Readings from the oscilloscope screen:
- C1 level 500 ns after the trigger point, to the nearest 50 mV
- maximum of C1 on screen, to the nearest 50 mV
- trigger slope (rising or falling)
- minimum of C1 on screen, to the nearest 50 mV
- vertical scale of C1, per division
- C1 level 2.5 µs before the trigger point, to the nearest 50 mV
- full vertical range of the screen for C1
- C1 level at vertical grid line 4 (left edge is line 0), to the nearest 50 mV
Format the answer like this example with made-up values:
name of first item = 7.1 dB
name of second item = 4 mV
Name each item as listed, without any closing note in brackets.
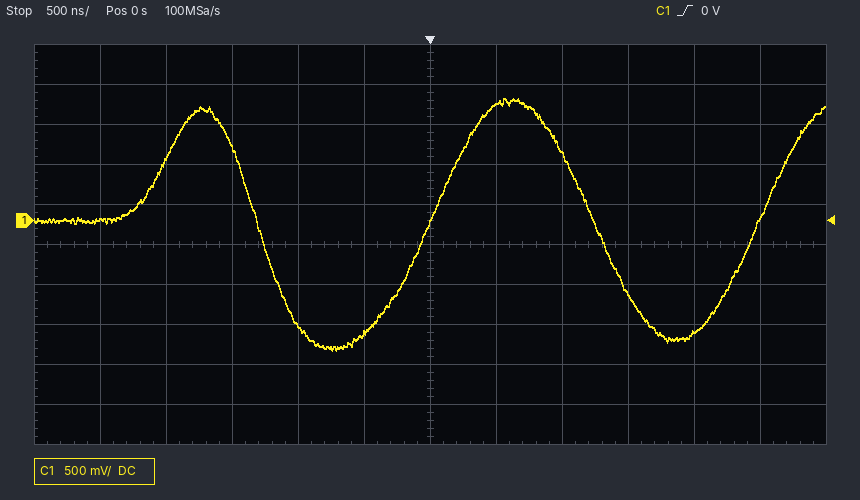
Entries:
C1 level 500 ns after the trigger point, to the nearest 50 mV = 1.45 V
maximum of C1 on screen, to the nearest 50 mV = 1.50 V
trigger slope = rising
minimum of C1 on screen, to the nearest 50 mV = -1.60 V
vertical scale of C1, per division = 500 mV
C1 level 2.5 µs before the trigger point, to the nearest 50 mV = 0 mV
full vertical range of the screen for C1 = 5 V
C1 level at vertical grid line 4 (left edge is line 0), to the nearest 50 mV = -1.30 V
